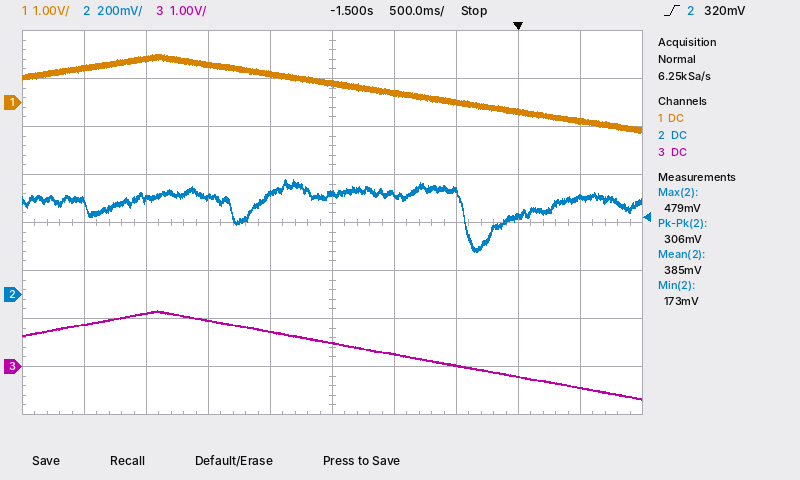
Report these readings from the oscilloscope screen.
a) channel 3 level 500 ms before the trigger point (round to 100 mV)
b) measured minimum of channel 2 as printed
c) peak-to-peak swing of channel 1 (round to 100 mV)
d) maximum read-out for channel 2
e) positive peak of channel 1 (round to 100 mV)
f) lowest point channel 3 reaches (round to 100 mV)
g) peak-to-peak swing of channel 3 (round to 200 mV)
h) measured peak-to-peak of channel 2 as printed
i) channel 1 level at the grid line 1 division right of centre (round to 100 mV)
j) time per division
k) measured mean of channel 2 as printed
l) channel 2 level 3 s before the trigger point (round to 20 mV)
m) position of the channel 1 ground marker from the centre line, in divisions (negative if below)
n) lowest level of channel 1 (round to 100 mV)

0.0 V
173 mV
1.6 V
479 mV
1.0 V
-700 mV
1.8 V
306 mV
200 mV
500 ms
385 mV
400 mV
+2.5 div
-600 mV
